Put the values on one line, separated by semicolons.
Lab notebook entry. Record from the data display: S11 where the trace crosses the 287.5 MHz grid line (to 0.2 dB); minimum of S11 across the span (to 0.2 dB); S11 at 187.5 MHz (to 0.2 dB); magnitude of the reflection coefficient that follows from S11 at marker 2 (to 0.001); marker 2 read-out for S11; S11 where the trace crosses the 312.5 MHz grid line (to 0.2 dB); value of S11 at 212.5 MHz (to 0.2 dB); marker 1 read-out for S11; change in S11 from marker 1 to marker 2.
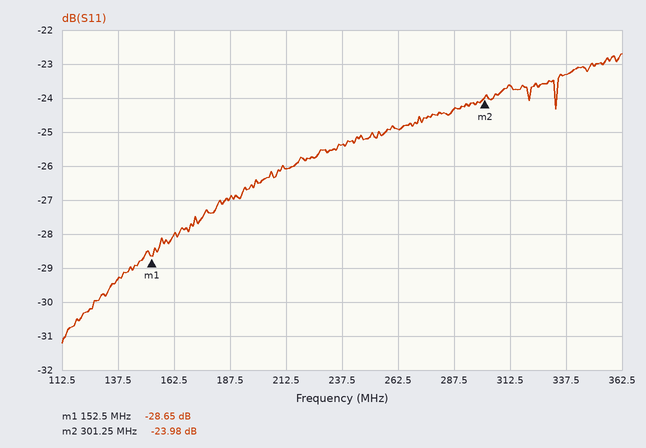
-24.4 dB; -31.2 dB; -27.0 dB; 0.063; -23.98 dB; -23.6 dB; -26.0 dB; -28.65 dB; 4.67 dB
